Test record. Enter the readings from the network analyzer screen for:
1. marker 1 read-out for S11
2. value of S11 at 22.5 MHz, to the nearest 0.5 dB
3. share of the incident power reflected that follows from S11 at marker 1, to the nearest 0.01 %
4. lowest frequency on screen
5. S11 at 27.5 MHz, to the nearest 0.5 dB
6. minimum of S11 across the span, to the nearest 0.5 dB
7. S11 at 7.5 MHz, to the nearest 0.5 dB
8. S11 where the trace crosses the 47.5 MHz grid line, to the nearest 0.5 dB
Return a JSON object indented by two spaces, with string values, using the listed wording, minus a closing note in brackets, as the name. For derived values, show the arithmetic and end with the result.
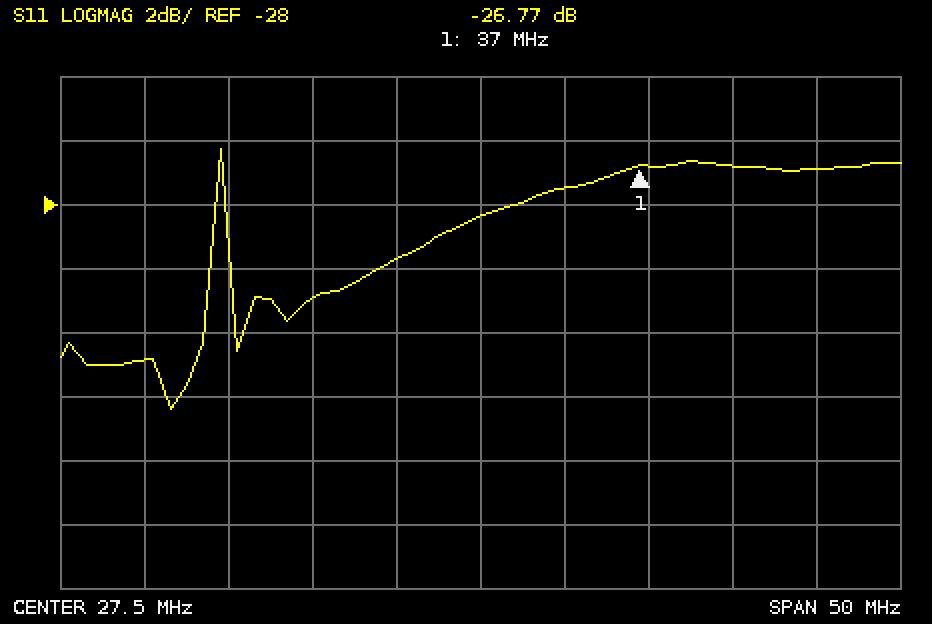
{
  "marker 1 read-out for S11": "-26.77 dB",
  "value of S11 at 22.5 MHz, to the nearest 0.5 dB": "-29.5 dB",
  "share of the incident power reflected that follows from S11 at marker 1, to the nearest 0.01 %": "10^(-26.77/10) ≈ 0.21 %",
  "lowest frequency on screen": "2.5 MHz",
  "S11 at 27.5 MHz, to the nearest 0.5 dB": "-28.5 dB",
  "minimum of S11 across the span, to the nearest 0.5 dB": "-34.5 dB",
  "S11 at 7.5 MHz, to the nearest 0.5 dB": "-33.0 dB",
  "S11 where the trace crosses the 47.5 MHz grid line, to the nearest 0.5 dB": "-27.0 dB"
}
